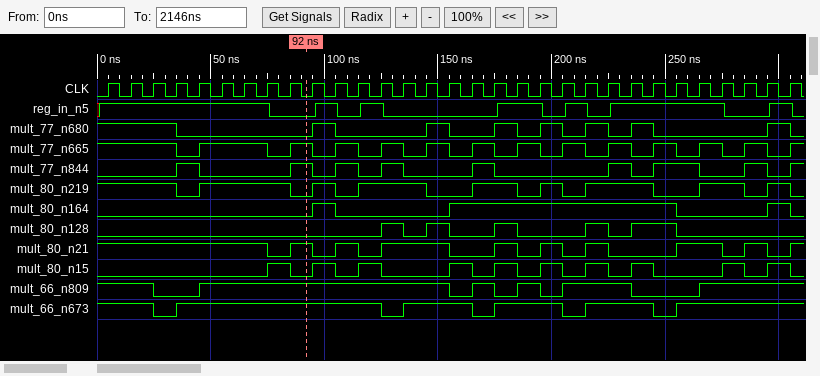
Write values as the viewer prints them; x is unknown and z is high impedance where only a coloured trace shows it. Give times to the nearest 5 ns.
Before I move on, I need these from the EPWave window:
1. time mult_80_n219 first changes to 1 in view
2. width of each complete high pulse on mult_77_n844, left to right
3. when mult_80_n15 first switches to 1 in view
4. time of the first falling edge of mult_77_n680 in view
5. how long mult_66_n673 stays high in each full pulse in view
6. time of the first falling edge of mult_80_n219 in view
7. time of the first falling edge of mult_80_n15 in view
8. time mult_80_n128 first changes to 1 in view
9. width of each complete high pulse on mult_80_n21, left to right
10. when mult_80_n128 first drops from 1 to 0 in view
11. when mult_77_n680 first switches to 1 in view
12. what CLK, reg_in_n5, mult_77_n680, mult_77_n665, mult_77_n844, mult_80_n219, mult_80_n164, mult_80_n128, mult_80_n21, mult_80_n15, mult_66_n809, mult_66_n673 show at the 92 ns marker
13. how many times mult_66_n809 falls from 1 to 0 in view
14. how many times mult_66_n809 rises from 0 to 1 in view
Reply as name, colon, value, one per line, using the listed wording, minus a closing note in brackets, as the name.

time mult_80_n219 first changes to 1 in view: 45 ns
width of each complete high pulse on mult_77_n844, left to right: 10 ns, 10 ns, 10 ns, 10 ns, 10 ns, 10 ns, 20 ns, 10 ns
when mult_80_n15 first switches to 1 in view: 75 ns
time of the first falling edge of mult_77_n680 in view: 35 ns
how long mult_66_n673 stays high in each full pulse in view: 90 ns, 30 ns, 30 ns, 30 ns
time of the first falling edge of mult_80_n219 in view: 35 ns
time of the first falling edge of mult_80_n15 in view: 85 ns
time mult_80_n128 first changes to 1 in view: 125 ns
width of each complete high pulse on mult_80_n21, left to right: 10 ns, 10 ns, 30 ns, 10 ns, 10 ns, 10 ns, 20 ns, 10 ns
when mult_80_n128 first drops from 1 to 0 in view: 135 ns
when mult_77_n680 first switches to 1 in view: 95 ns
what CLK, reg_in_n5, mult_77_n680, mult_77_n665, mult_77_n844, mult_80_n219, mult_80_n164, mult_80_n128, mult_80_n21, mult_80_n15, mult_66_n809, mult_66_n673 show at the 92 ns marker: CLK=0, reg_in_n5=0, mult_77_n680=0, mult_77_n665=1, mult_77_n844=1, mult_80_n219=0, mult_80_n164=0, mult_80_n128=0, mult_80_n21=1, mult_80_n15=0, mult_66_n809=1, mult_66_n673=1
how many times mult_66_n809 falls from 1 to 0 in view: 5
how many times mult_66_n809 rises from 0 to 1 in view: 5
